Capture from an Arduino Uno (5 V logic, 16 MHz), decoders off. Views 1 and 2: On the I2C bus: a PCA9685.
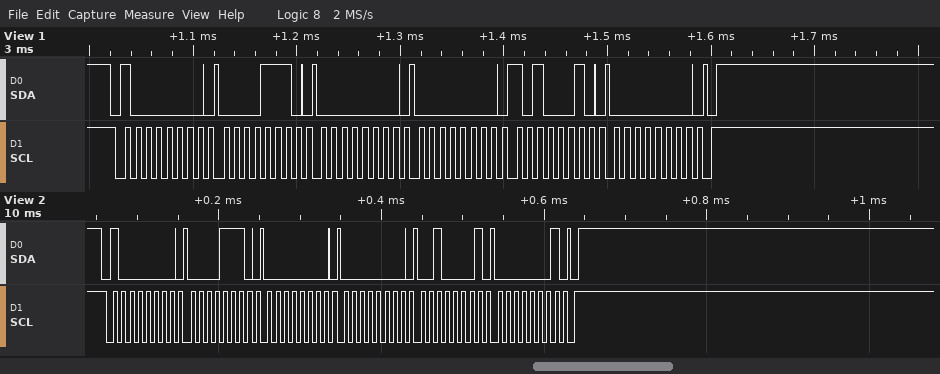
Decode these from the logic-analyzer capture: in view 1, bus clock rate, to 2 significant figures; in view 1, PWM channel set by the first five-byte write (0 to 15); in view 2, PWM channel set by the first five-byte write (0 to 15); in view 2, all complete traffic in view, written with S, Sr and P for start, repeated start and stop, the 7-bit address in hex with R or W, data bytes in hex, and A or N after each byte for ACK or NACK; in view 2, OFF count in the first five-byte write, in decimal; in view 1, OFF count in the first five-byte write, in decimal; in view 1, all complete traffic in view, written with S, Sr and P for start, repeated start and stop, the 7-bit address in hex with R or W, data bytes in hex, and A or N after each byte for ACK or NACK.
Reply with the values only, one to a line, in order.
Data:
100 kHz
2
2
S 40W A 0E A 00 A 00 A 21 A 01 A P
289
162
S 40W A 0E A 00 A 00 A A2 A 00 A P
